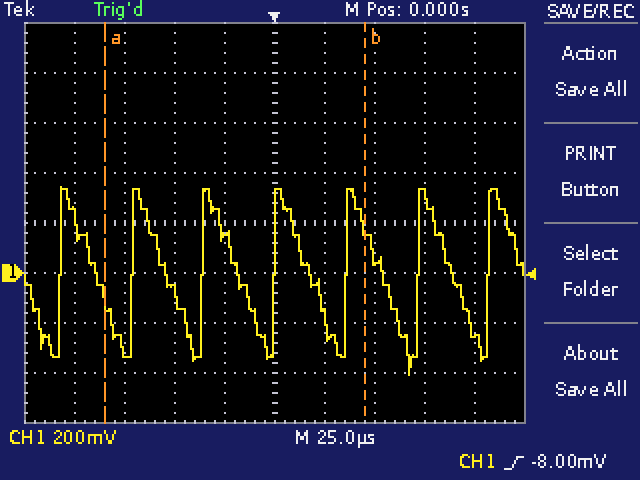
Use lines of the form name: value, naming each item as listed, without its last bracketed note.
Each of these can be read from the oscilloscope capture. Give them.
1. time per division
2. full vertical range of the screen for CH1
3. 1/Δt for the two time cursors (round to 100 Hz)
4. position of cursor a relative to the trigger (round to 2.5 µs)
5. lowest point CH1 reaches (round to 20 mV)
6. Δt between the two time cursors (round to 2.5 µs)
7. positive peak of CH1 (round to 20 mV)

time per division: 25 µs
full vertical range of the screen for CH1: 1.6 V
1/Δt for the two time cursors: 7.7 kHz
position of cursor a relative to the trigger: -85.0 µs
lowest point CH1 reaches: -400 mV
Δt between the two time cursors: 130.0 µs
positive peak of CH1: 340 mV
